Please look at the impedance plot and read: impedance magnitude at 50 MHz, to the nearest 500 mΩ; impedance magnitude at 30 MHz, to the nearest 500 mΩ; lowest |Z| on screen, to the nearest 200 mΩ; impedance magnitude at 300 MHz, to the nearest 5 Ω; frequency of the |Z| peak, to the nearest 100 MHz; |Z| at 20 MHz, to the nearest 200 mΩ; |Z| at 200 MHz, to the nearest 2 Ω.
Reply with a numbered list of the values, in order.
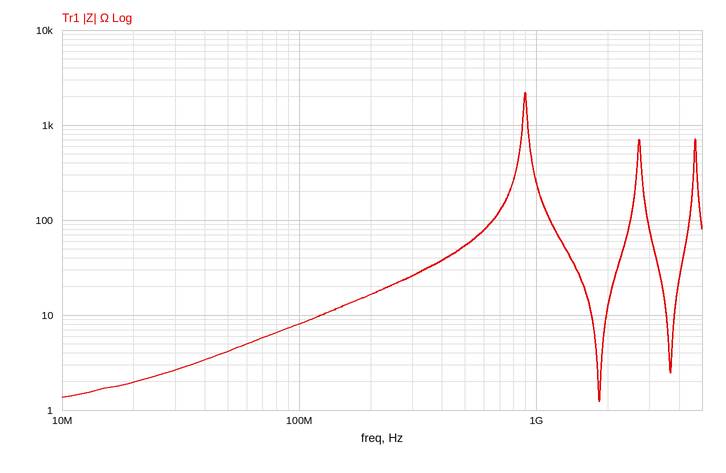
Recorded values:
1. 4.0 Ω
2. 2.5 Ω
3. 1.2 Ω
4. 25 Ω
5. 900 MHz
6. 2.0 Ω
7. 16 Ω
